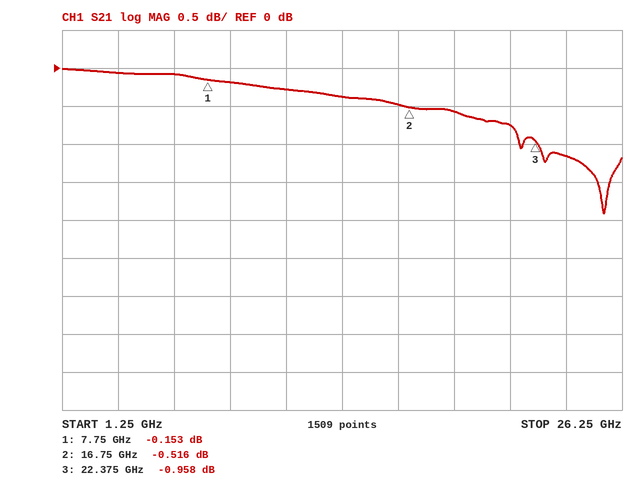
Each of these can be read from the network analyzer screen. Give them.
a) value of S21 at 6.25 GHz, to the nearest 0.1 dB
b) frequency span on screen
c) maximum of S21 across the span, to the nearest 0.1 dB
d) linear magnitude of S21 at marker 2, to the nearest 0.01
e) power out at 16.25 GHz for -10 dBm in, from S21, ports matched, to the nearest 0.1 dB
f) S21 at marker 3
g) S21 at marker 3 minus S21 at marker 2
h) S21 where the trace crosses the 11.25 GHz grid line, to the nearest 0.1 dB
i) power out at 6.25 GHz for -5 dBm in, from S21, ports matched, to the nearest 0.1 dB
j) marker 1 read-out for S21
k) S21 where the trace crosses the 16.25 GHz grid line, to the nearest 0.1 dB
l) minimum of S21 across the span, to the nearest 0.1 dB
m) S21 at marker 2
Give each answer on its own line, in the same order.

-0.1 dB
25 GHz
0.0 dB
0.94
-10.5 dBm
-0.958 dB
-0.442 dB
-0.3 dB
-5.1 dBm
-0.153 dB
-0.5 dB
-1.9 dB
-0.516 dB
